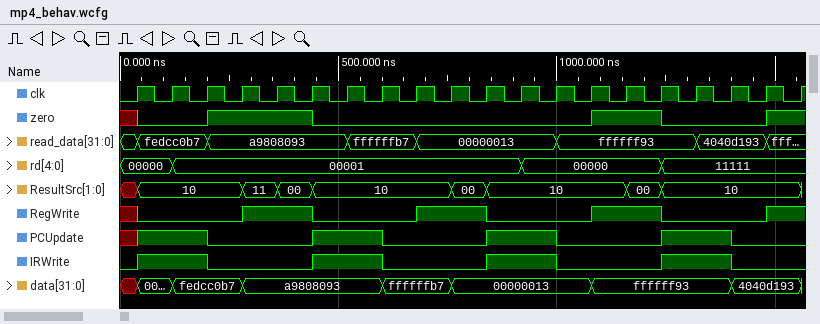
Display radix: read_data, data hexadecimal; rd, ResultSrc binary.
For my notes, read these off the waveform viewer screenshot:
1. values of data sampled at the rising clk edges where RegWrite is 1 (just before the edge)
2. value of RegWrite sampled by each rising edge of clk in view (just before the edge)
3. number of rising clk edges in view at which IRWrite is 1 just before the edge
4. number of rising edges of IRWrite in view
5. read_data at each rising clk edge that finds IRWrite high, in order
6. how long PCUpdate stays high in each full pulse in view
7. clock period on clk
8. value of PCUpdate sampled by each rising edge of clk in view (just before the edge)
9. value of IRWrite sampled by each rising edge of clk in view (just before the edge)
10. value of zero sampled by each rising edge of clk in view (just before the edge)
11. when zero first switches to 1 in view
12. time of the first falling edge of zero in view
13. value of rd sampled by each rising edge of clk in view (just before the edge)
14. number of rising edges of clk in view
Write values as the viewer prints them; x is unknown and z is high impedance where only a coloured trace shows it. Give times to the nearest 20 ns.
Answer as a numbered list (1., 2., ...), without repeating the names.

1. a9808093, a9808093, ffffffb7, 00000013, ffffff93, ffffff93, 4040d193
2. x 0 0 0 1 1 0 0 0 1 1 0 0 0 1 1 0 0 0 1
3. 8
4. 4
5. fedcc0b7, fedcc0b7, a9808093, ffffffb7, 00000013, 00000013, ffffff93, 4040d193
6. 160 ns, 160 ns, 160 ns
7. 80 ns
8. x 1 1 0 0 0 1 1 0 0 0 1 1 0 0 0 1 1 0 0
9. 0 1 1 0 0 0 1 1 0 0 0 1 1 0 0 0 1 1 0 0
10. x 0 0 1 1 1 0 0 0 0 0 0 0 0 1 1 0 0 0 1
11. 200 ns
12. 440 ns
13. 00000, 00000, 00001, 00001, 00001, 00001, 00001, 00001, 00001, 00001, 00001, 00001, 00000, 00000, 00000, 00000, 11111, 11111, 11111, 11111
14. 20
